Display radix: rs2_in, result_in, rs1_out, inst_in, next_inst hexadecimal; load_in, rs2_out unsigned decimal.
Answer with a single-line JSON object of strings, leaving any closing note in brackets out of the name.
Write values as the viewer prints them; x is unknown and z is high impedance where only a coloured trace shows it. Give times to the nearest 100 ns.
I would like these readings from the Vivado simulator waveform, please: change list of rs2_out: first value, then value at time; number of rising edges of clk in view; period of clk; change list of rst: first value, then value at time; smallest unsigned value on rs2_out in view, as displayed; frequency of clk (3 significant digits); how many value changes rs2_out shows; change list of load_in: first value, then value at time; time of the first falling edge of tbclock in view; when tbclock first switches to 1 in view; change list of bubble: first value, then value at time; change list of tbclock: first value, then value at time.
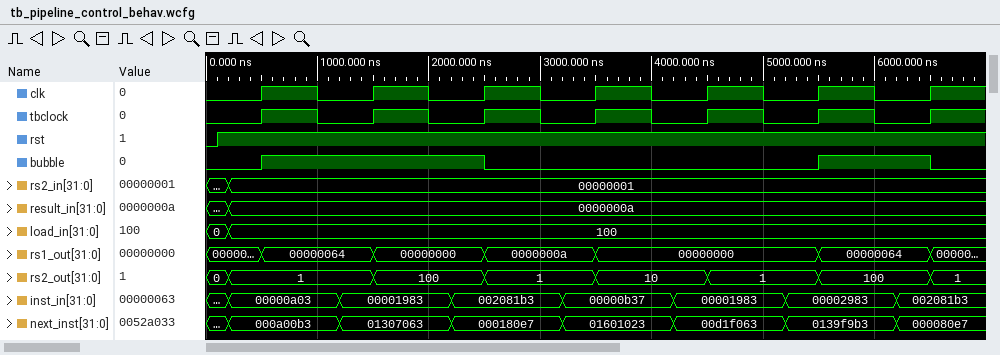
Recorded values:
{"change list of rs2_out: first value, then value at time": "0, 1 at 200 ns, 100 at 1500 ns, 1 at 2500 ns, 10 at 3500 ns, 1 at 4500 ns, 100 at 5500 ns, 1 at 6500 ns", "number of rising edges of clk in view": "7", "period of clk": "1000 ns", "change list of rst: first value, then value at time": "0, 1 at 100 ns", "smallest unsigned value on rs2_out in view, as displayed": "0", "frequency of clk": "1.00 MHz", "how many value changes rs2_out shows": "7", "change list of load_in: first value, then value at time": "0, 100 at 200 ns", "time of the first falling edge of tbclock in view": "1000 ns", "when tbclock first switches to 1 in view": "500 ns", "change list of bubble: first value, then value at time": "0, 1 at 500 ns, 0 at 2500 ns, 1 at 5500 ns, 0 at 6500 ns", "change list of tbclock: first value, then value at time": "0, 1 at 500 ns, 0 at 1000 ns, 1 at 1500 ns, 0 at 2000 ns, 1 at 2500 ns, 0 at 3000 ns, 1 at 3500 ns, 0 at 4000 ns, 1 at 4500 ns, 0 at 5000 ns, 1 at 5500 ns, 0 at 6000 ns, 1 at 6500 ns"}
